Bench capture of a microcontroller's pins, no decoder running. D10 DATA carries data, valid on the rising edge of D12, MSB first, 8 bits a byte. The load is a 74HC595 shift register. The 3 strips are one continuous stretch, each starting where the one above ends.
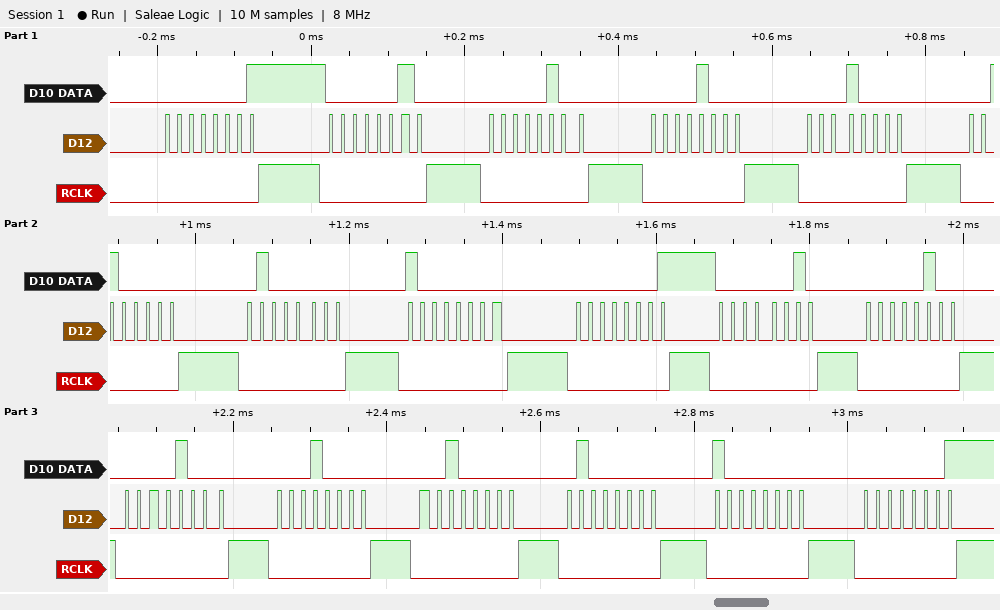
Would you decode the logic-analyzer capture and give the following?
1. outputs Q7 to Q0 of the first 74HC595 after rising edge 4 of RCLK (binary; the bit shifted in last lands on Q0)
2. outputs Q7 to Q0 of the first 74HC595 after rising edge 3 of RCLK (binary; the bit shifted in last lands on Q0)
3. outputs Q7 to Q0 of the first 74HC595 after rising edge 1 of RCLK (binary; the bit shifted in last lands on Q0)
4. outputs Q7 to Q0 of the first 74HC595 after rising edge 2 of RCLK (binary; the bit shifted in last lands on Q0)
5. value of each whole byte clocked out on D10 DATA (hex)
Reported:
00001000
00000100
00000001
00000010
0x01 0x02 0x04 0x08 0x10 0x20 0x40 0x80 0x01 0x02 0x04 0x08 0x10 0x20 0x40 0x80 0x01
